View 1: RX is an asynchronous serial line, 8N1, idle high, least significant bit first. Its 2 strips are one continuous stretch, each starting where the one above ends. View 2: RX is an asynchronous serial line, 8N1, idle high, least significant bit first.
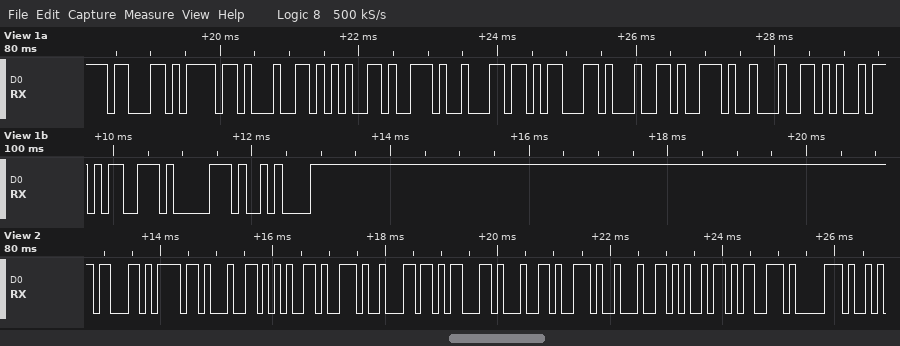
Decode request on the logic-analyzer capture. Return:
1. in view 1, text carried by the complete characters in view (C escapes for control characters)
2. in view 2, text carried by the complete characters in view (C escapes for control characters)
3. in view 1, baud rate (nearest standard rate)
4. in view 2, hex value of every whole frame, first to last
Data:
"code.lcd.disp\n"
"code.lcd.disp"
9600 baud
63 6F 64 65 2E 6C 63 64 2E 64 69 73 70
